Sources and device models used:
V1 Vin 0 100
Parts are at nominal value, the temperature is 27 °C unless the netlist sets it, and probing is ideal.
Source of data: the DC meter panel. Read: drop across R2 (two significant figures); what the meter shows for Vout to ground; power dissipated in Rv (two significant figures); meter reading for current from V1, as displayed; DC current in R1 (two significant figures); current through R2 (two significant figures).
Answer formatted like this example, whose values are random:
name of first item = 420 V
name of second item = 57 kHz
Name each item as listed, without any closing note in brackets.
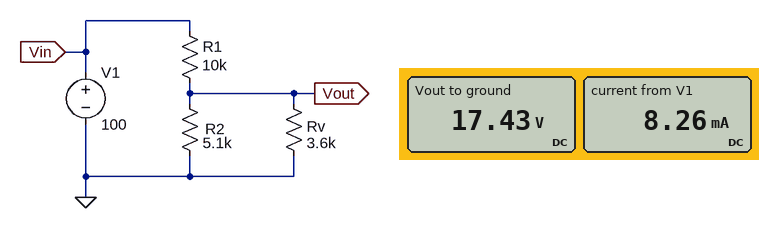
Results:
drop across R2 = 17 V
what the meter shows for Vout to ground = 17.43 V
power dissipated in Rv = 84 mW
meter reading for current from V1, as displayed = 8.26 mA
DC current in R1 = 8.3 mA
current through R2 = 3.4 mA
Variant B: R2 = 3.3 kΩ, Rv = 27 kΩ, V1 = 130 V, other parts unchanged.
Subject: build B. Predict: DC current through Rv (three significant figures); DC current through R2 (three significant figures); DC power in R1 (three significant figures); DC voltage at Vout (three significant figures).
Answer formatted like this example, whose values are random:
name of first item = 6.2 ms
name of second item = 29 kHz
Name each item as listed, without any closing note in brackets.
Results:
DC current through Rv = 1.09 mA
DC current through R2 = 8.95 mA
DC power in R1 = 1.01 W
DC voltage at Vout = 29.5 V
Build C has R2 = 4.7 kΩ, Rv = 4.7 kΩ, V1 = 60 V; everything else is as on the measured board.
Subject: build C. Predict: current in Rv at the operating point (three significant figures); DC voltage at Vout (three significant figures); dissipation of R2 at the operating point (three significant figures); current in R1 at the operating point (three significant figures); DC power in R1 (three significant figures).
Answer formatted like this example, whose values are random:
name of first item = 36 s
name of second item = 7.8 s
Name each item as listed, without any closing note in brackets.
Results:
current in Rv at the operating point = 2.43 mA
DC voltage at Vout = 11.4 V
dissipation of R2 at the operating point = 27.7 mW
current in R1 at the operating point = 4.86 mA
DC power in R1 = 236 mW
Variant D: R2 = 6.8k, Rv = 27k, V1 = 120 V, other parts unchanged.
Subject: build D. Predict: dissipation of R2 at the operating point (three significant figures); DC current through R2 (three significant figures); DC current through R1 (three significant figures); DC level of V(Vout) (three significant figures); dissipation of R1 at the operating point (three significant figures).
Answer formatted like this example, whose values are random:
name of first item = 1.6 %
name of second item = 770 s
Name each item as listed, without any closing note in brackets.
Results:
dissipation of R2 at the operating point = 262 mW
DC current through R2 = 6.21 mA
DC current through R1 = 7.78 mA
DC level of V(Vout) = 42.2 V
dissipation of R1 at the operating point = 605 mW
